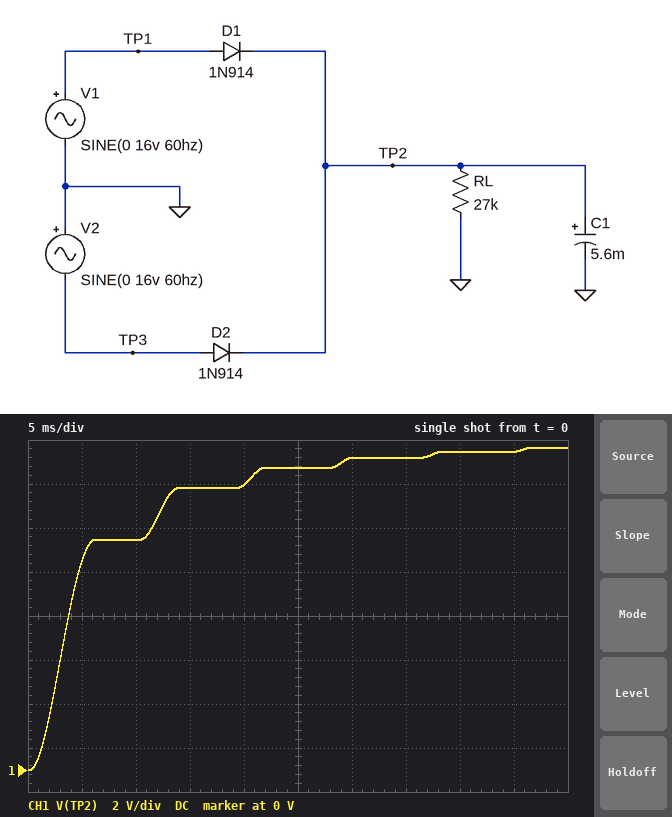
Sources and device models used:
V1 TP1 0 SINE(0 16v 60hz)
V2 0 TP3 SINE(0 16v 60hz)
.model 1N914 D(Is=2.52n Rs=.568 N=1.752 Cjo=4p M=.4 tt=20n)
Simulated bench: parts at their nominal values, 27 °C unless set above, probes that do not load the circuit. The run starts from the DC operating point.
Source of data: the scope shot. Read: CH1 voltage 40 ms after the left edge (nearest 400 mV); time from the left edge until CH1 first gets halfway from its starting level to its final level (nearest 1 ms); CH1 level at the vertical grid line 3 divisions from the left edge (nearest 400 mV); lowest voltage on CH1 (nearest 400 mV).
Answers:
14.4 V
4 ms
12.8 V
0 V
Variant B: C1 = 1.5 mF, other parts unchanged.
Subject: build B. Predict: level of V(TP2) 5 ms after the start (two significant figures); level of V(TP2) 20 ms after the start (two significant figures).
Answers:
14 V
15 V
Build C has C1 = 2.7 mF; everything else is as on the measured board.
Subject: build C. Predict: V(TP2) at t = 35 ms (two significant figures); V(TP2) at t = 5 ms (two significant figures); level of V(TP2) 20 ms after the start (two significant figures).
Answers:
15 V
13 V
14 V
